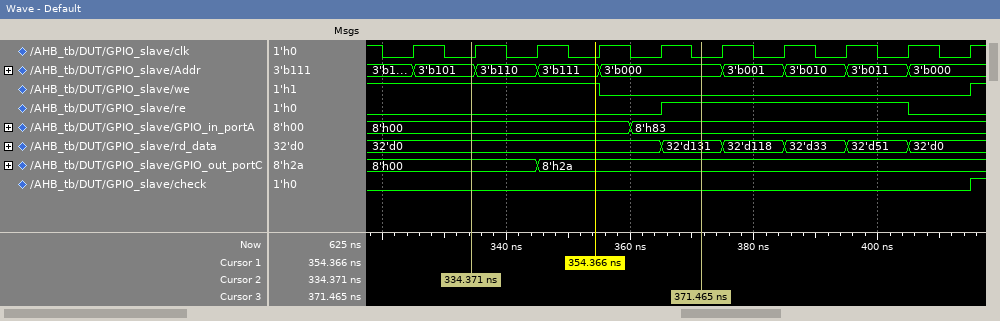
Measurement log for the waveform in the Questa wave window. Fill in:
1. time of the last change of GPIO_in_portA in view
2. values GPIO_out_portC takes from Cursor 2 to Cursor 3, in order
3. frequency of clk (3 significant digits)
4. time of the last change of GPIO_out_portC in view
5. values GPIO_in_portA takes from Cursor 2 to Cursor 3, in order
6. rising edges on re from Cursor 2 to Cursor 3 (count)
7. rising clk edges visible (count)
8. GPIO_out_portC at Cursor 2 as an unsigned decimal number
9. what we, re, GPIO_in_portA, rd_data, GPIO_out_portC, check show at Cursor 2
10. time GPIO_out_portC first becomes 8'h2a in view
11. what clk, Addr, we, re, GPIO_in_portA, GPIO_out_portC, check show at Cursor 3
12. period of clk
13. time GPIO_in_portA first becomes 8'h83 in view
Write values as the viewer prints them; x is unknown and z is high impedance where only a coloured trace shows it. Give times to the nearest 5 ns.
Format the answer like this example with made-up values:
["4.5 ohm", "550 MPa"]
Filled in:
["360 ns", "8'h00, 8'h2a", "100 MHz", "345 ns", "8'h00, 8'h83", "1", "10", "0", "we=1, re=0, GPIO_in_portA=8'h00, rd_data=32'd0, GPIO_out_portC=8'h00, check=0", "345 ns", "clk=0, Addr=3'b000, we=0, re=1, GPIO_in_portA=8'h83, GPIO_out_portC=8'h2a, check=0", "10 ns", "360 ns"]
